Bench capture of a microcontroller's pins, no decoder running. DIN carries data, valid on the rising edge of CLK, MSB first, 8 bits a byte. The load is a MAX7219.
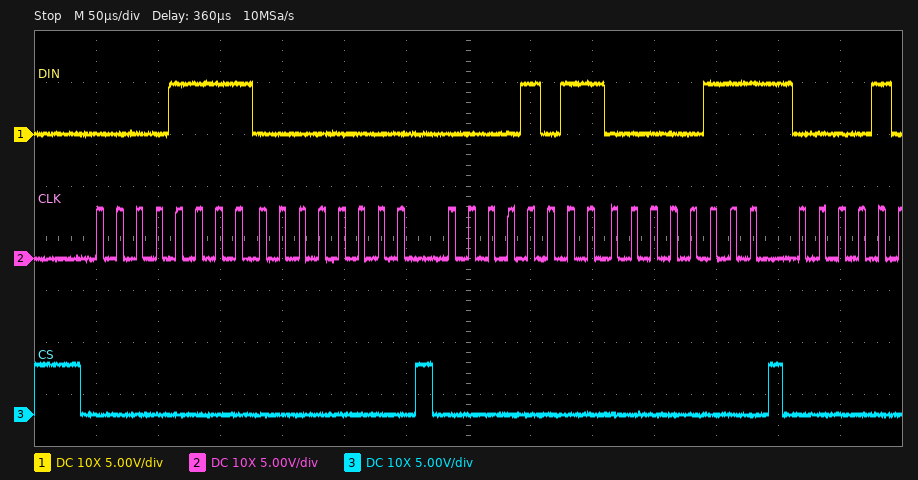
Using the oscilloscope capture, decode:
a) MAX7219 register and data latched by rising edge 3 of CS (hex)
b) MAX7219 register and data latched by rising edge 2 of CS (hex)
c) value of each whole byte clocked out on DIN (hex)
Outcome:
register 0xB, data 0x07
register 0xF, data 0x00
0F 00 0B 07
